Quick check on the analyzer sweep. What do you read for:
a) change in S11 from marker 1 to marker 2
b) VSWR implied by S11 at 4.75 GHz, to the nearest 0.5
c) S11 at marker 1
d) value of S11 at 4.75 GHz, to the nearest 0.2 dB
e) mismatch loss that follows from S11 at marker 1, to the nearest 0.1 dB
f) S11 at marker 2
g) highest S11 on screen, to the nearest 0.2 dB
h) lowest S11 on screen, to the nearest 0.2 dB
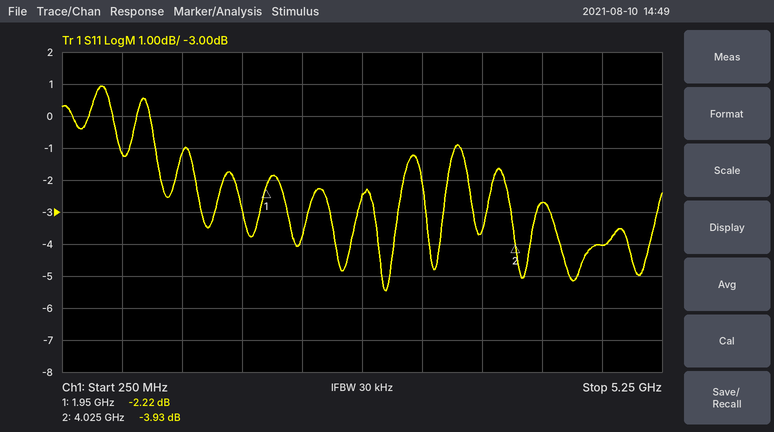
-1.71 dB
4.5
-2.22 dB
-4.0 dB
4.0 dB
-3.93 dB
1.0 dB
-5.4 dB
